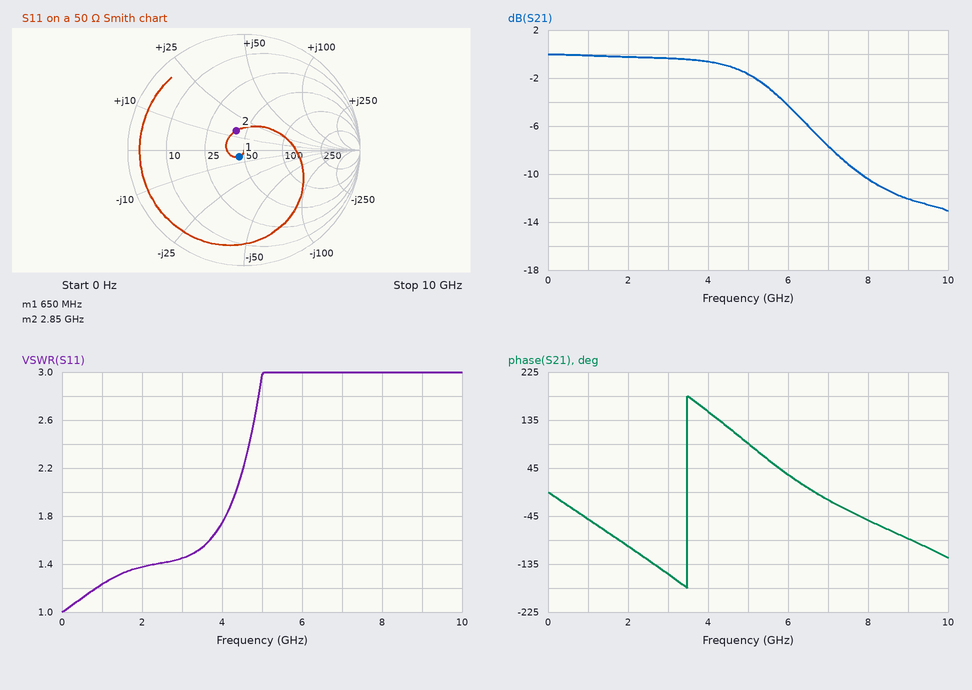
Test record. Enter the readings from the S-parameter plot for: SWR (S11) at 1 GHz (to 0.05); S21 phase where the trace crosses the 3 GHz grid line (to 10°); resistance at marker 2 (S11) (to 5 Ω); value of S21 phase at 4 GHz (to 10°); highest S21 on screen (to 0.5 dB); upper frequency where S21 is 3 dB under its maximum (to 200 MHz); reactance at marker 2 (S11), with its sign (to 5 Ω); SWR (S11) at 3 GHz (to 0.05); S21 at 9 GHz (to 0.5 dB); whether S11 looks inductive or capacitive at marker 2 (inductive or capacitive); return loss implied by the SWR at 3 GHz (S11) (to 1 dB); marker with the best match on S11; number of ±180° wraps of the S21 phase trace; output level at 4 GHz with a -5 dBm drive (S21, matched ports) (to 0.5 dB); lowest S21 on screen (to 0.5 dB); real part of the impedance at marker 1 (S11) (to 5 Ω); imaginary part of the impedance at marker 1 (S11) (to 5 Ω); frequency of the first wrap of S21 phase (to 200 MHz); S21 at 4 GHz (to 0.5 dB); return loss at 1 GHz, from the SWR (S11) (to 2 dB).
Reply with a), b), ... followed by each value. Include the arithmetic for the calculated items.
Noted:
a) 1.25
b) -150°
c) 40 Ω
d) 150°
e) 0.0 dB
f) 5.6 GHz
g) +15 Ω
h) 1.45
i) -12.0 dB
j) inductive
k) −20 log10((1.45 − 1)/(1.45 + 1)) ≈ 15 dB
l) marker 1
m) 1
n) -5 dBm + (-0.5 dB) = -5.5 dBm
o) -13.0 dB
p) 45 Ω
q) -5 Ω
r) 3.4 GHz
s) -0.5 dB
t) −20 log10((1.25 − 1)/(1.25 + 1)) ≈ 19.1 dB, so 20 dB to the nearest 2 dB
